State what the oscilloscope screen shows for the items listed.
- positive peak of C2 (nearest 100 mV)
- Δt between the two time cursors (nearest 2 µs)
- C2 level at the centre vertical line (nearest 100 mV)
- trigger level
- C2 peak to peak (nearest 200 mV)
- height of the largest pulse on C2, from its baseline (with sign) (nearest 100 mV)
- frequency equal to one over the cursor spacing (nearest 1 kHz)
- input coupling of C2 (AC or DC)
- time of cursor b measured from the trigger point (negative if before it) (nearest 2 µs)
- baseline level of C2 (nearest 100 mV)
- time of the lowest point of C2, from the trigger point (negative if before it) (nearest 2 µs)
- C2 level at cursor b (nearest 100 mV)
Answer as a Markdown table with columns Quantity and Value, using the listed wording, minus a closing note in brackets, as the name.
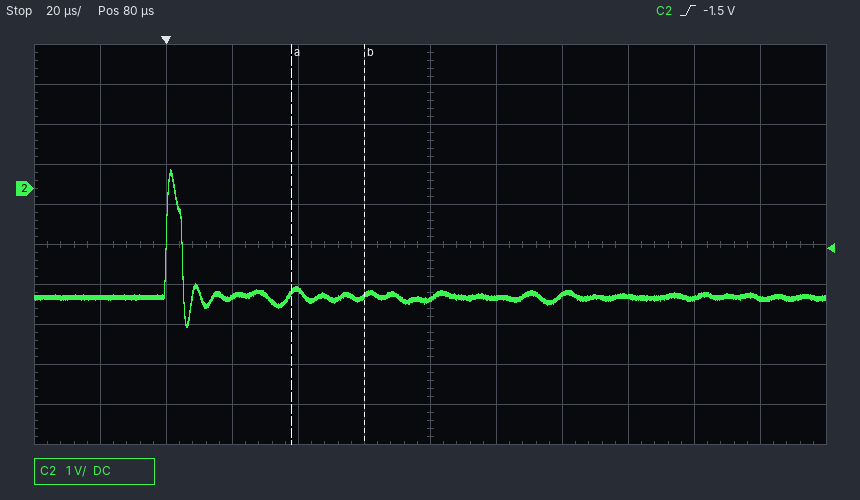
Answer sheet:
| Quantity | Value |
|---|---|
| positive peak of C2 | 500 mV |
| Δt between the two time cursors | 22 µs |
| C2 level at the centre vertical line | -2.8 V |
| trigger level | -1.5 V |
| C2 peak to peak | 4.0 V |
| height of the largest pulse on C2, from its baseline (with sign) | +3.2 V |
| frequency equal to one over the cursor spacing | 45 kHz |
| input coupling of C2 | DC |
| time of cursor b measured from the trigger point (negative if before it) | +60 µs |
| baseline level of C2 | -2.7 V |
| time of the lowest point of C2, from the trigger point (negative if before it) | +6 µs |
| C2 level at cursor b | -2.7 V |
